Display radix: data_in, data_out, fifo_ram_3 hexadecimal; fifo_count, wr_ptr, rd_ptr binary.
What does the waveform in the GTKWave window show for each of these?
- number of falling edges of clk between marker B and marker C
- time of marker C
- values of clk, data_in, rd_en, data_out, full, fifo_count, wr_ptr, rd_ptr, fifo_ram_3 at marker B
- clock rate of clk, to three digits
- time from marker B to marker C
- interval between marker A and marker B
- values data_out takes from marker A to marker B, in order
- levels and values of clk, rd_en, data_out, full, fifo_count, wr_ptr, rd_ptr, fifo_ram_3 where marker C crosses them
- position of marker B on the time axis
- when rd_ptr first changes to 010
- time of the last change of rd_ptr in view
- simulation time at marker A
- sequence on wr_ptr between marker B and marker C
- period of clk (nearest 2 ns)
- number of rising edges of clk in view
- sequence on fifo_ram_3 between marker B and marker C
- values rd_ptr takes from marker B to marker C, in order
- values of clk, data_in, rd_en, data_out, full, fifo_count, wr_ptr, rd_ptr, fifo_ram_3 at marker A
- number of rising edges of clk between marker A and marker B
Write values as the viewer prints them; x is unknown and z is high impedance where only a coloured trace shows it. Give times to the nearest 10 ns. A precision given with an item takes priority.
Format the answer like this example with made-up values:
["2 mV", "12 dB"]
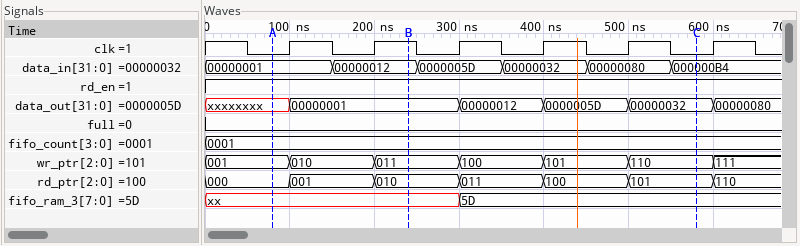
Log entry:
["4", "580 ns", "clk=1, data_in=00000012, rd_en=1, data_out=00000001, full=0, fifo_count=0001, wr_ptr=011, rd_ptr=010, fifo_ram_3=xx", "10.0 MHz", "340 ns", "160 ns", "xxxxxxxx, 00000001", "clk=0, rd_en=1, data_out=00000032, full=0, fifo_count=0001, wr_ptr=110, rd_ptr=101, fifo_ram_3=5D", "240 ns", "200 ns", "600 ns", "80 ns", "011, 100, 101, 110", "100 ns", "6", "xx, 5D", "010, 011, 100, 101", "clk=0, data_in=00000001, rd_en=1, data_out=xxxxxxxx, full=0, fifo_count=0001, wr_ptr=001, rd_ptr=000, fifo_ram_3=xx", "2"]
